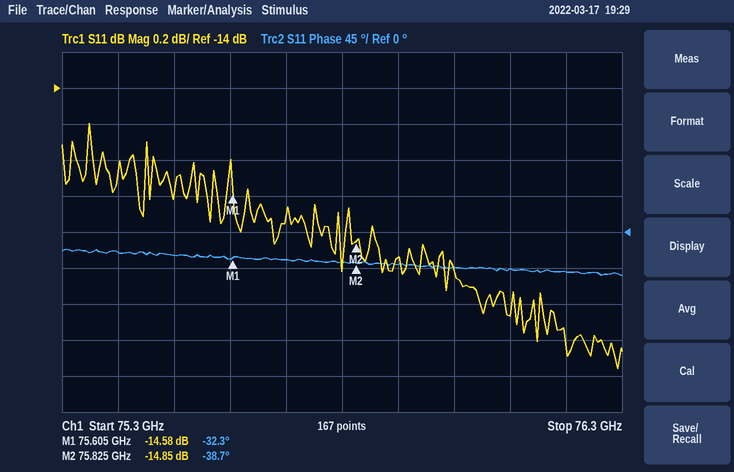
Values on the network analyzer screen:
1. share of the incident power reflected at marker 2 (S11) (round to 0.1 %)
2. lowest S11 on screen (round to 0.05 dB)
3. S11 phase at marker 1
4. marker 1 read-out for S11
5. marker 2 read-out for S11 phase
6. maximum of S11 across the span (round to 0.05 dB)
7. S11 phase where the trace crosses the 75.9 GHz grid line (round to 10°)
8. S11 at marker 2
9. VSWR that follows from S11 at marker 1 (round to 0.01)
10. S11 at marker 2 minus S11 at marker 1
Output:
3.3 %
-15.55 dB
-32.3°
-14.58 dB
-38.7°
-14.20 dB
-40°
-14.85 dB
1.46
-0.27 dB
